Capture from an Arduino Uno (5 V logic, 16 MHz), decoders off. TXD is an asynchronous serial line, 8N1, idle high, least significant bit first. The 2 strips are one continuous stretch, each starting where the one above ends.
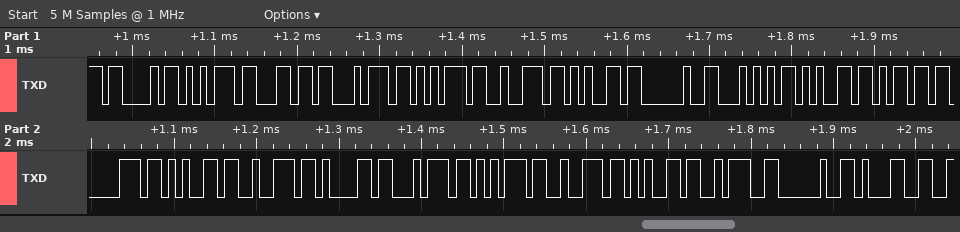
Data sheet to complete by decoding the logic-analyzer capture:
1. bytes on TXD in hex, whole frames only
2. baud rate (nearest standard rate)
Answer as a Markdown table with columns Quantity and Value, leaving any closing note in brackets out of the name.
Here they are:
| Quantity | Value |
|---|---|
| bytes on TXD in hex, whole frames only | 43 75 6C 74 75 72 65 20 54 65 6D 70 65 72 61 74 75 72 65 3A 20 31 |
| baud rate | 115200 baud |
